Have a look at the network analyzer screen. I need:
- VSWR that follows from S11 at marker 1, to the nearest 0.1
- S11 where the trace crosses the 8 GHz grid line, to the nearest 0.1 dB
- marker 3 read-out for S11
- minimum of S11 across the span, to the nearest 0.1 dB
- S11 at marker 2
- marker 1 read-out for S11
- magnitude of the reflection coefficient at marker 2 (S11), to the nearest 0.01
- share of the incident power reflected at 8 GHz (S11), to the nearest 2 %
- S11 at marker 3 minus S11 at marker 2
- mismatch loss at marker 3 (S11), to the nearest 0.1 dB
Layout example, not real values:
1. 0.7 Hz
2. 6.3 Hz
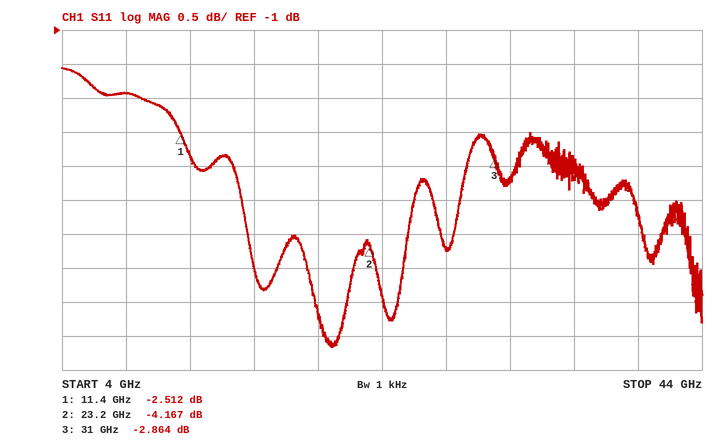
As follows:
1. 7.0
2. -1.9 dB
3. -2.864 dB
4. -5.7 dB
5. -4.167 dB
6. -2.512 dB
7. 0.62
8. 64 %
9. 1.303 dB
10. 3.2 dB
